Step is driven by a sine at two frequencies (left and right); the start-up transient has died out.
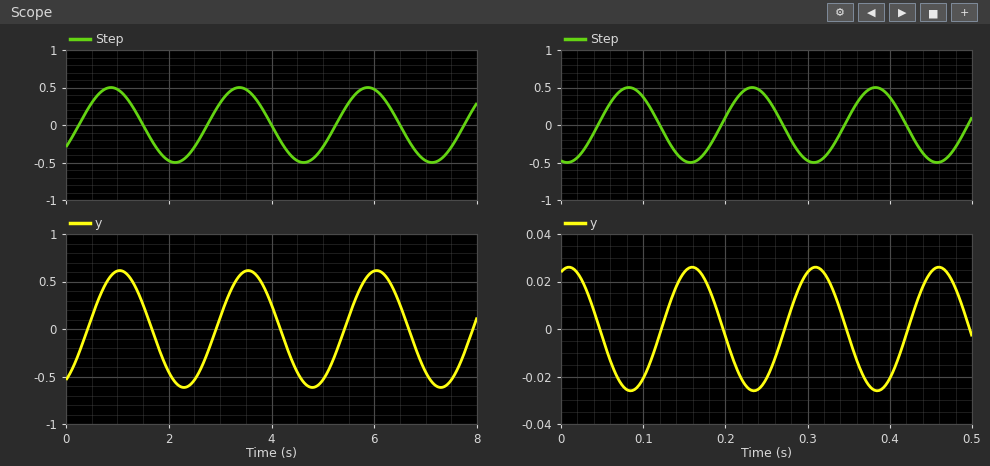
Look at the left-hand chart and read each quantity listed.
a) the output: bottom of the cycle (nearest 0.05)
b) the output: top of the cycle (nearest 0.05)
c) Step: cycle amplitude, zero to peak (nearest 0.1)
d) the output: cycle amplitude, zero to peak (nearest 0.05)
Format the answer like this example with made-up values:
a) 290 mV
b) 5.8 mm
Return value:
a) -0.60
b) 0.60
c) 0.5
d) 0.60
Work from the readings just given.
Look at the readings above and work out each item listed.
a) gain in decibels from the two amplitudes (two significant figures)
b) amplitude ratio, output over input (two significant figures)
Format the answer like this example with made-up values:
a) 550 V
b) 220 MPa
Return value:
a) 1.6 dB
b) 1.2
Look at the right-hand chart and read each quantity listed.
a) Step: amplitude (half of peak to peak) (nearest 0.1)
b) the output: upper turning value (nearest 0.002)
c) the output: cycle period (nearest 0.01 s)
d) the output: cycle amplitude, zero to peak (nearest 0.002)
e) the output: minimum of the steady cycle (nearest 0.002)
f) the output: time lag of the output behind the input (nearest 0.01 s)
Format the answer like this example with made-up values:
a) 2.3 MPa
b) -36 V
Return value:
a) 0.5
b) 0.026
c) 0.15 s
d) 0.026
e) -0.026
f) 0.08 s
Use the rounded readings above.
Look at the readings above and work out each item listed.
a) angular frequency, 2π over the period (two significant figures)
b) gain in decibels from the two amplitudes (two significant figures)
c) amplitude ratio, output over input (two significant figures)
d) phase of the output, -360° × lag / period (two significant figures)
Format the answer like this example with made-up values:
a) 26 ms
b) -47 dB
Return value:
a) 42 rad/s
b) -26 dB
c) 0.052
d) -190°
